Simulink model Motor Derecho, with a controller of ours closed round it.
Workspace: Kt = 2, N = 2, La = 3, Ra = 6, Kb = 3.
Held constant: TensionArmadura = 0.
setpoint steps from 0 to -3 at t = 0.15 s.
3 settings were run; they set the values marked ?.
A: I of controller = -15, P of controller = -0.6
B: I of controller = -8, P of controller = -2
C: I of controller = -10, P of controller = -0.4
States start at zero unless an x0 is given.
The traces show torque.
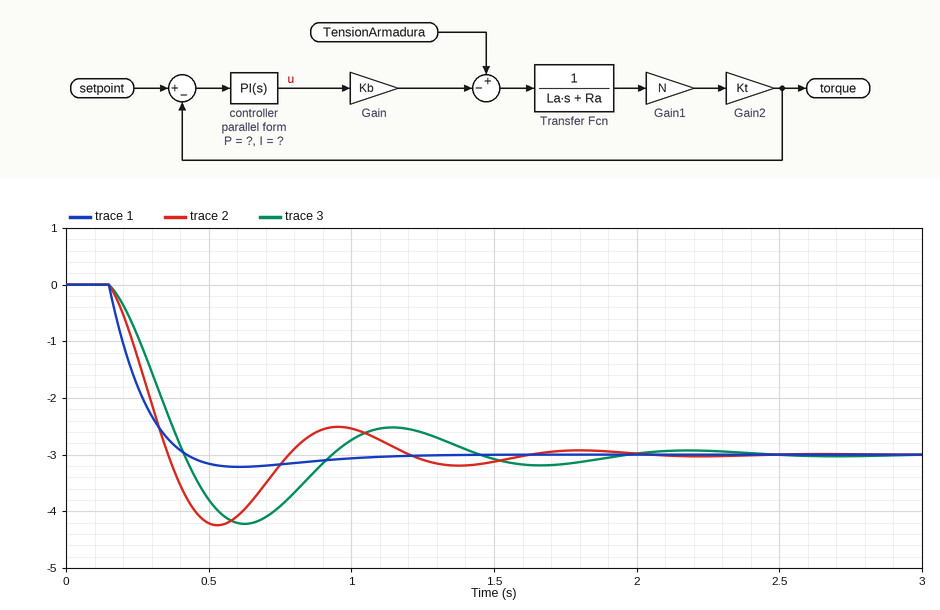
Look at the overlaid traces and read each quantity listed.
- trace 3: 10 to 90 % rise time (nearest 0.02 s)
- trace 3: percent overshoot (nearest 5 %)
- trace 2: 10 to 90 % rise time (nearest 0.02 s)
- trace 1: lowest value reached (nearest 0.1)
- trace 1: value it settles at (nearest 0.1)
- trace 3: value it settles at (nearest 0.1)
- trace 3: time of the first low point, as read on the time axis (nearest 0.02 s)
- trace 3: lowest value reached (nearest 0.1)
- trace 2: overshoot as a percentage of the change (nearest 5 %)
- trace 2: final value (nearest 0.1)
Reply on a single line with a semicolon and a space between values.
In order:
0.20 s; 40 %; 0.16 s; -3.2; -3.0; -3.0; 0.62 s; -4.2; 40 %; -3.0
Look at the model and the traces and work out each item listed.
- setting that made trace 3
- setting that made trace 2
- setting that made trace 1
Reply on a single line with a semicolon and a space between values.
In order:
C; A; B
